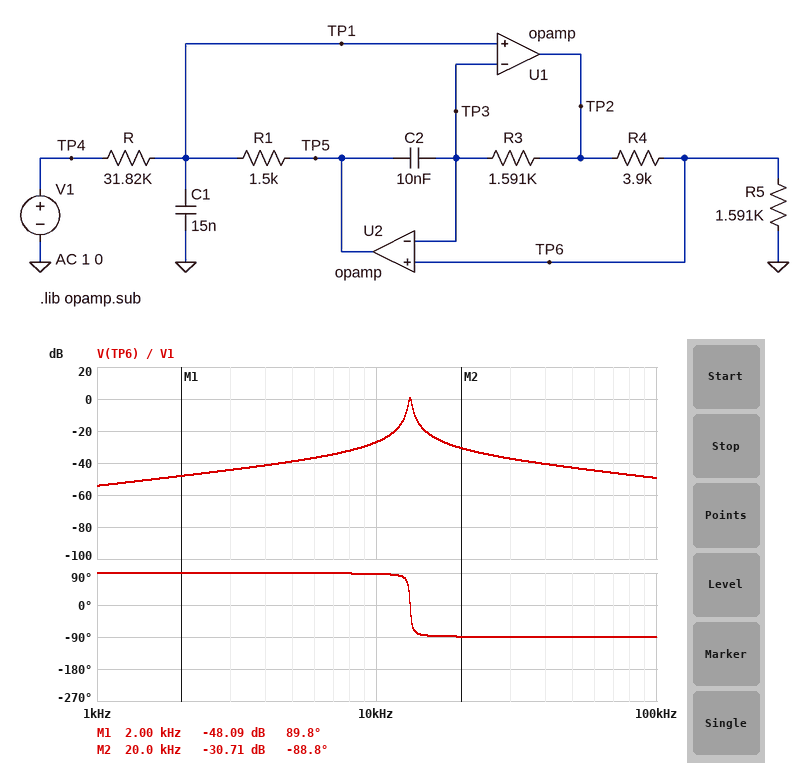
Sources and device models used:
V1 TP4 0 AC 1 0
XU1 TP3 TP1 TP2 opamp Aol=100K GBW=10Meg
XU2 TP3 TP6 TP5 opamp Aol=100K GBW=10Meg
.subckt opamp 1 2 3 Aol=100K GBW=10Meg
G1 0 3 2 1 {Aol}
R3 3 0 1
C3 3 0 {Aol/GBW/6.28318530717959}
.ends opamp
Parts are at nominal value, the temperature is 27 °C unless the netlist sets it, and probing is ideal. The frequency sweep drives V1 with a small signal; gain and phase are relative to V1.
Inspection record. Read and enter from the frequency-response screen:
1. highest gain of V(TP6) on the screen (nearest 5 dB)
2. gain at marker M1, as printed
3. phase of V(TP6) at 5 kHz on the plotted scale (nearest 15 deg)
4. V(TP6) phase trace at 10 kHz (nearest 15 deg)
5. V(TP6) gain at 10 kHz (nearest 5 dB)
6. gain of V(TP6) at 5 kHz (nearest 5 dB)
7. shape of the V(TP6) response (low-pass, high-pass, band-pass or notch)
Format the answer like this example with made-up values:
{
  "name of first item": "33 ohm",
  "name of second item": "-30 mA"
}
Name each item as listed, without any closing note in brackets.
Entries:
{
  "highest gain of V(TP6) on the screen": "0 dB",
  "gain at marker M1, as printed": "-48.09 dB",
  "phase of V(TP6) at 5 kHz on the plotted scale": "90 deg",
  "V(TP6) phase trace at 10 kHz": "90 deg",
  "V(TP6) gain at 10 kHz": "-25 dB",
  "gain of V(TP6) at 5 kHz": "-40 dB",
  "shape of the V(TP6) response": "band-pass"
}
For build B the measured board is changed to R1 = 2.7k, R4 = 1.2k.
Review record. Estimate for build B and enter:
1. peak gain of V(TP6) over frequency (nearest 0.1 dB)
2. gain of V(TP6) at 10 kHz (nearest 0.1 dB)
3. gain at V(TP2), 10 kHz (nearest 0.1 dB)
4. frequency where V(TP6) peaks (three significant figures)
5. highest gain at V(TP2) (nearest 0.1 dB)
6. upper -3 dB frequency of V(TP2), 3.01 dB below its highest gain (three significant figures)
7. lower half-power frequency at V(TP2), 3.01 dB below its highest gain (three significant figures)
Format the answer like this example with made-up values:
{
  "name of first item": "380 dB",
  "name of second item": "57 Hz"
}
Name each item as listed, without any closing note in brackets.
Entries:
{
  "peak gain of V(TP6) over frequency": "-0.1 dB",
  "gain of V(TP6) at 10 kHz": "-26.5 dB",
  "gain at V(TP2), 10 kHz": "-21.6 dB",
  "frequency where V(TP6) peaks": "5.44 kHz",
  "highest gain at V(TP2)": "4.8 dB",
  "upper -3 dB frequency of V(TP2), 3.01 dB below its highest gain": "5.61 kHz",
  "lower half-power frequency at V(TP2), 3.01 dB below its highest gain": "5.27 kHz"
}
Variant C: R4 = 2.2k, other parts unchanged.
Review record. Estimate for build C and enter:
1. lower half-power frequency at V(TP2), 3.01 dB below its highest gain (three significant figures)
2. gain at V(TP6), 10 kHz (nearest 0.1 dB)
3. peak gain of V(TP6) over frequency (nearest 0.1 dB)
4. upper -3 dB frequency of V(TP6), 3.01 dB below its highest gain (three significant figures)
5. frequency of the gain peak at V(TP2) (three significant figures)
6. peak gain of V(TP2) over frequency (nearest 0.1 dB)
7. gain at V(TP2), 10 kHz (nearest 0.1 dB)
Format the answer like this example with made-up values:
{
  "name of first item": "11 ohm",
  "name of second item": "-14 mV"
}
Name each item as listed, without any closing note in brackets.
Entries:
{
  "lower half-power frequency at V(TP2), 3.01 dB below its highest gain": "9.71 kHz",
  "gain at V(TP6), 10 kHz": "-1.9 dB",
  "peak gain of V(TP6) over frequency": "0.1 dB",
  "upper -3 dB frequency of V(TP6), 3.01 dB below its highest gain": "10.0 kHz",
  "frequency of the gain peak at V(TP2)": "9.87 kHz",
  "peak gain of V(TP2) over frequency": "7.7 dB",
  "gain at V(TP2), 10 kHz": "5.6 dB"
}
